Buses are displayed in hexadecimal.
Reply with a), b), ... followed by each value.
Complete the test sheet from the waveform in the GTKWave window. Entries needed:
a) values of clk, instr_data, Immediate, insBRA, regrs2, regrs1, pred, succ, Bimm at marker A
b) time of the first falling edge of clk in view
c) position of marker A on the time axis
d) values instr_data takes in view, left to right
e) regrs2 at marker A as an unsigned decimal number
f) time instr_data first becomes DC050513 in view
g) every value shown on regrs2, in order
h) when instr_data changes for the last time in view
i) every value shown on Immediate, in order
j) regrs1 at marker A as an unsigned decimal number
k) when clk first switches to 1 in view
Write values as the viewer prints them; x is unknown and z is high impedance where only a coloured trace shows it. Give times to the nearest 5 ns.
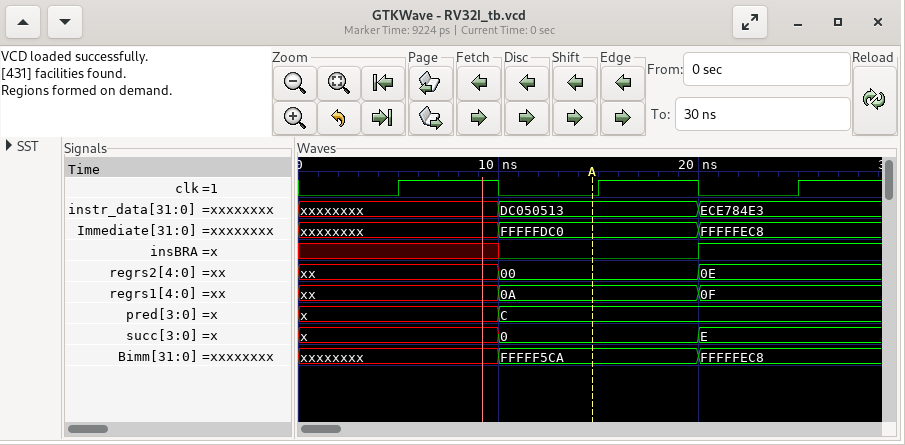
a) clk=0, instr_data=DC050513, Immediate=FFFFFDC0, insBRA=0, regrs2=00, regrs1=0A, pred=C, succ=0, Bimm=FFFFF5CA
b) 10 ns
c) 15 ns
d) xxxxxxxx, DC050513, ECE784E3
e) 0
f) 10 ns
g) xx, 00, 0E
h) 20 ns
i) xxxxxxxx, FFFFFDC0, FFFFFEC8
j) 10
k) 5 ns
